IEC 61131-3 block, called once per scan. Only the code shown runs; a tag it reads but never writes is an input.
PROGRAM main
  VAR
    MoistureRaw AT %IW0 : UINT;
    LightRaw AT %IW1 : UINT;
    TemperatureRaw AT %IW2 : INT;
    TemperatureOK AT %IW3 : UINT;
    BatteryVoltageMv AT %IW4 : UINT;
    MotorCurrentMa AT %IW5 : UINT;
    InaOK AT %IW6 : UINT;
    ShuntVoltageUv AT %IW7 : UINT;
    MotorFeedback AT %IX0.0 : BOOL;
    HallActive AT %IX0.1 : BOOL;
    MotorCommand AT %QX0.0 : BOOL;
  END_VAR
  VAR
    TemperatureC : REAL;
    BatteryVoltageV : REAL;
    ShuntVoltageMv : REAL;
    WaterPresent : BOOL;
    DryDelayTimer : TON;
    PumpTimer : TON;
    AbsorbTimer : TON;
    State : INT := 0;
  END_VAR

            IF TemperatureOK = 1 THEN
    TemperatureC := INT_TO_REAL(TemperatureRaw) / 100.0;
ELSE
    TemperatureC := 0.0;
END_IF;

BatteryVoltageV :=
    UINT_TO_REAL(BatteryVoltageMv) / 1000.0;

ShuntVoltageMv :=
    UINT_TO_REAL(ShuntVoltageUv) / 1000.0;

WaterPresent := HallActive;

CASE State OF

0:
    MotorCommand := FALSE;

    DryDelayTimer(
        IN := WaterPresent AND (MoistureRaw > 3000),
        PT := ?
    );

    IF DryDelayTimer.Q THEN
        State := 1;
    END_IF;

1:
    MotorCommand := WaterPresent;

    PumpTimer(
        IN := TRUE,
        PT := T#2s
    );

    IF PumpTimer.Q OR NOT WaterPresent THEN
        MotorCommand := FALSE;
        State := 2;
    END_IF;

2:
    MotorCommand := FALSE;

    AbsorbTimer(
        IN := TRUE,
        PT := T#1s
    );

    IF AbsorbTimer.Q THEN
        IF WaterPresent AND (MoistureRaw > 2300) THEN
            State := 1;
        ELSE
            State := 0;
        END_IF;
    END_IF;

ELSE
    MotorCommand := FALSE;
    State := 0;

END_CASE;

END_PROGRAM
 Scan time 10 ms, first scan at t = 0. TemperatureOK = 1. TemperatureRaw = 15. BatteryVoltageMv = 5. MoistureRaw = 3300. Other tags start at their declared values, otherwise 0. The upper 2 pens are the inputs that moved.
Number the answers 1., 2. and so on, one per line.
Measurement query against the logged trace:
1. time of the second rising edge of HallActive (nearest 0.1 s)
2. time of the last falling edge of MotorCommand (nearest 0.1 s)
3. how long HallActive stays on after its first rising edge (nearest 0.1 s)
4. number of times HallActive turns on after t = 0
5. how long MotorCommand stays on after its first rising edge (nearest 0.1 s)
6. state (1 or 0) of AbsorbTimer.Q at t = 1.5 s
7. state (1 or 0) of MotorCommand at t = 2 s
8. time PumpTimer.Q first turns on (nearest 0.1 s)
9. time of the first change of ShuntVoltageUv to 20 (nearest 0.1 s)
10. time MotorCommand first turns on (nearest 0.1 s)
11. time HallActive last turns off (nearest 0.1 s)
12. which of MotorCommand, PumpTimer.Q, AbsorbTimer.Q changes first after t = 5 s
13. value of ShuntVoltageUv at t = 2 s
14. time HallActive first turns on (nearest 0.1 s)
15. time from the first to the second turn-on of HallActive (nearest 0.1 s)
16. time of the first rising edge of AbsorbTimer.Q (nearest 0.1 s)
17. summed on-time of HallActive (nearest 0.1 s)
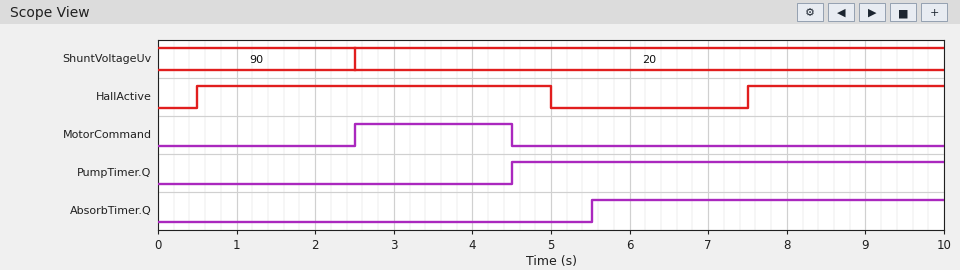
1. 7.5 s
2. 4.5 s
3. 4.5 s
4. 2
5. 2.0 s
6. 0
7. 0
8. 4.5 s
9. 2.5 s
10. 2.5 s
11. 5.0 s
12. AbsorbTimer.Q
13. 90
14. 0.5 s
15. 7.0 s
16. 5.5 s
17. 7.0 s
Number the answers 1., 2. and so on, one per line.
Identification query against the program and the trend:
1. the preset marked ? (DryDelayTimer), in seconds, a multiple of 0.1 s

1. 2.0 s
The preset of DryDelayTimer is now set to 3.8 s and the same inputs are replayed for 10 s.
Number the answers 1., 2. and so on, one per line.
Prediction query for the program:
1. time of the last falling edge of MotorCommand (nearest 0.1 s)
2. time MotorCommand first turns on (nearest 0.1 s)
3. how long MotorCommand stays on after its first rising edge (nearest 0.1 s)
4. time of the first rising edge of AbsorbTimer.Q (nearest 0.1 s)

1. 5.0 s
2. 4.3 s
3. 0.7 s
4. 6.0 s
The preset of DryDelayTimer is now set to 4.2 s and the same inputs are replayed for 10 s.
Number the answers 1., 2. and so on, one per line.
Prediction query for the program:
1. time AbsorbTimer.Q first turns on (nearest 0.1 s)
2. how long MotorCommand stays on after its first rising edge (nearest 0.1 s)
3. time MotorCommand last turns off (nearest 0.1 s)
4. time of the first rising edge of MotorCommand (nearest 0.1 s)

1. 6.0 s
2. 0.3 s
3. 5.0 s
4. 4.7 s
